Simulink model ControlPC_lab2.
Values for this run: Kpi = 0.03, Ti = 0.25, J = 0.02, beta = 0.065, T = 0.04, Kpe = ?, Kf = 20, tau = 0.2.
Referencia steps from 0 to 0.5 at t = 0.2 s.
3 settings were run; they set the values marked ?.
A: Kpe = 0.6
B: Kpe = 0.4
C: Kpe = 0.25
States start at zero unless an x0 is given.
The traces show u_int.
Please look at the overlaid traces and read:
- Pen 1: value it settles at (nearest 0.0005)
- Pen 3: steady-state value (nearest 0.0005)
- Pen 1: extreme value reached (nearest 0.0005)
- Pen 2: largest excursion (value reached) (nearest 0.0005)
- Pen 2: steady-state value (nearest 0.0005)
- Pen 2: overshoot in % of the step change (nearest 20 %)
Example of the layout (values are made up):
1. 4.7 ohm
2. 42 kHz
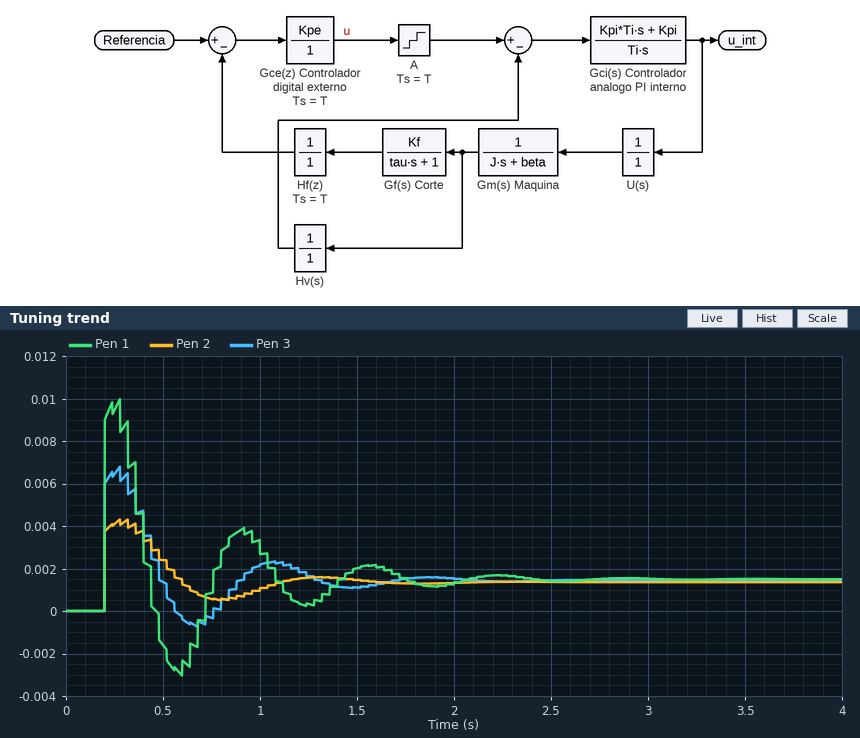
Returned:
1. 0.0015
2. 0.0015
3. 0.0100
4. 0.0045
5. 0.0015
6. 220 %
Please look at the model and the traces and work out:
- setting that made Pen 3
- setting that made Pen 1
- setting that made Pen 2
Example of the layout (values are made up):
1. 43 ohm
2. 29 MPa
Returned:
1. B
2. A
3. C
